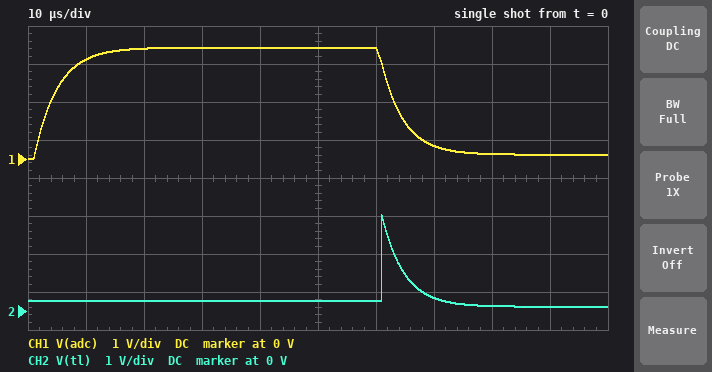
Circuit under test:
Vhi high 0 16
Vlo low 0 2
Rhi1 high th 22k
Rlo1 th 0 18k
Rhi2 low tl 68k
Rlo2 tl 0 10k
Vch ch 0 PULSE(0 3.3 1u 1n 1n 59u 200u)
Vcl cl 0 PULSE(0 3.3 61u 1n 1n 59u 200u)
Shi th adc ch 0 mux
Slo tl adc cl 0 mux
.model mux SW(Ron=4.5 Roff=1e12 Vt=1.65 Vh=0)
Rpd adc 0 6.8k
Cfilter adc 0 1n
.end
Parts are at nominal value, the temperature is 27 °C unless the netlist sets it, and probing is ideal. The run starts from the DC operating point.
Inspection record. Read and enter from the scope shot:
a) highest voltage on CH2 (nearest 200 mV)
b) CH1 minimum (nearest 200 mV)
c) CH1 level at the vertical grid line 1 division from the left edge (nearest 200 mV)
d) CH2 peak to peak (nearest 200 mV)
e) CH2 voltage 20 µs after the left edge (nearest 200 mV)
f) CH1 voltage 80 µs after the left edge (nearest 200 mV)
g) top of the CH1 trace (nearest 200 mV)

2.6 V
0 V
2.6 V
2.4 V
200 mV
200 mV
3.0 V
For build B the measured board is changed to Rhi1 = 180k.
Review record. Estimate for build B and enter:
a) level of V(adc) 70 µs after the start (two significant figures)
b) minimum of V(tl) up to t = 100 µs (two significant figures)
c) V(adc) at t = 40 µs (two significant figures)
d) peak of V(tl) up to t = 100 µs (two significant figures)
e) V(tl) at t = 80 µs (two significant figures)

140 mV
110 mV
430 mV
370 mV
110 mV
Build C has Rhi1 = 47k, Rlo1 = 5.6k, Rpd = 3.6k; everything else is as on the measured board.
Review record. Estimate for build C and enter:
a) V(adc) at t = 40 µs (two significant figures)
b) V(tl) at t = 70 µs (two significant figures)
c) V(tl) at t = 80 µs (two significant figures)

710 mV
89 mV
75 mV
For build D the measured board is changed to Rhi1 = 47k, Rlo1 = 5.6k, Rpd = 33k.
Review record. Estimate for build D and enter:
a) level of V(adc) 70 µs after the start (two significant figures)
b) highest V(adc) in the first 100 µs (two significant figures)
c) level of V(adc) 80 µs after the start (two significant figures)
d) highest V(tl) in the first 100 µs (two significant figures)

540 mV
1.5 V
280 mV
1.4 V
